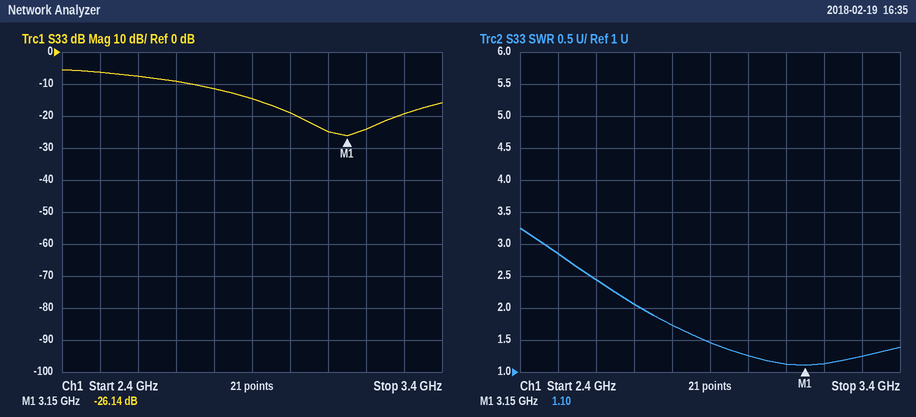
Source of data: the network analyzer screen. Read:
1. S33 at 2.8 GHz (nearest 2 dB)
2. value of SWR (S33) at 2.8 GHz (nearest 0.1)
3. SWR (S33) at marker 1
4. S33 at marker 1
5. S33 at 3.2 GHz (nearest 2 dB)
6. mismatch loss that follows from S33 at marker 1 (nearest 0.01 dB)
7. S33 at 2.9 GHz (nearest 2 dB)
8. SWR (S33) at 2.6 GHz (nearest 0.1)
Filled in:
-12 dB
1.7
1.10
-26.14 dB
-24 dB
0.01 dB
-14 dB
2.4
